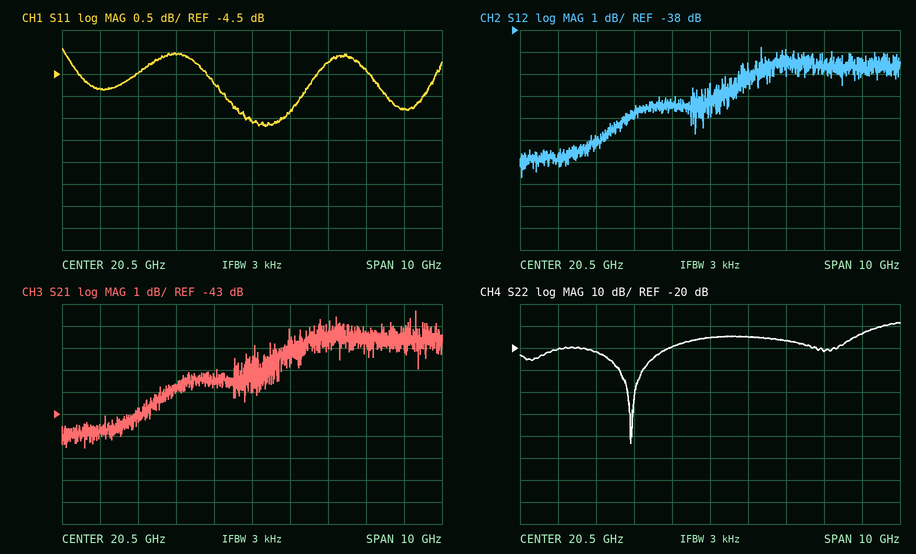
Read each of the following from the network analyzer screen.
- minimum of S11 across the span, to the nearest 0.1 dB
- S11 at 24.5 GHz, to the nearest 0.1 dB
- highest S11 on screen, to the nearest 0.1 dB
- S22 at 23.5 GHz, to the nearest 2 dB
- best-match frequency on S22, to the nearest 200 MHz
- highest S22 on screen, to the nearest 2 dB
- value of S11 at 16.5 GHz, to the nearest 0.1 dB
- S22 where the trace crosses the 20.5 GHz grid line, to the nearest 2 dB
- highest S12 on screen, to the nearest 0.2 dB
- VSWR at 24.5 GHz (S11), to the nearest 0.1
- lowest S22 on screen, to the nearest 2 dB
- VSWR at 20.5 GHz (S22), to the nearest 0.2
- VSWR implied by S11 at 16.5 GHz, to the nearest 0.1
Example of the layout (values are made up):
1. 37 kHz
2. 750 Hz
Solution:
1. -5.7 dB
2. -5.3 dB
3. -3.9 dB
4. -22 dB
5. 18.4 GHz
6. -8 dB
7. -4.8 dB
8. -16 dB
9. -38.8 dB
10. 3.4
11. -64 dB
12. 1.4
13. 3.7
